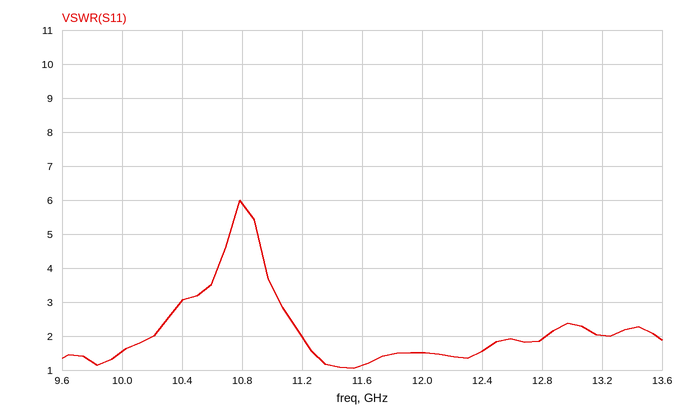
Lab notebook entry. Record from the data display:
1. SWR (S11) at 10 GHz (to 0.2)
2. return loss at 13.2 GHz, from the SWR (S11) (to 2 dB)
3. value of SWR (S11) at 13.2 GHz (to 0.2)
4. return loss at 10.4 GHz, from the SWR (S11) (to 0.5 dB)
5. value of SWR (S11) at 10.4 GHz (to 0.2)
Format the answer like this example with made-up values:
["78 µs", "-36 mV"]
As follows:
["1.6", "10 dB", "2.0", "6.0 dB", "3.0"]
